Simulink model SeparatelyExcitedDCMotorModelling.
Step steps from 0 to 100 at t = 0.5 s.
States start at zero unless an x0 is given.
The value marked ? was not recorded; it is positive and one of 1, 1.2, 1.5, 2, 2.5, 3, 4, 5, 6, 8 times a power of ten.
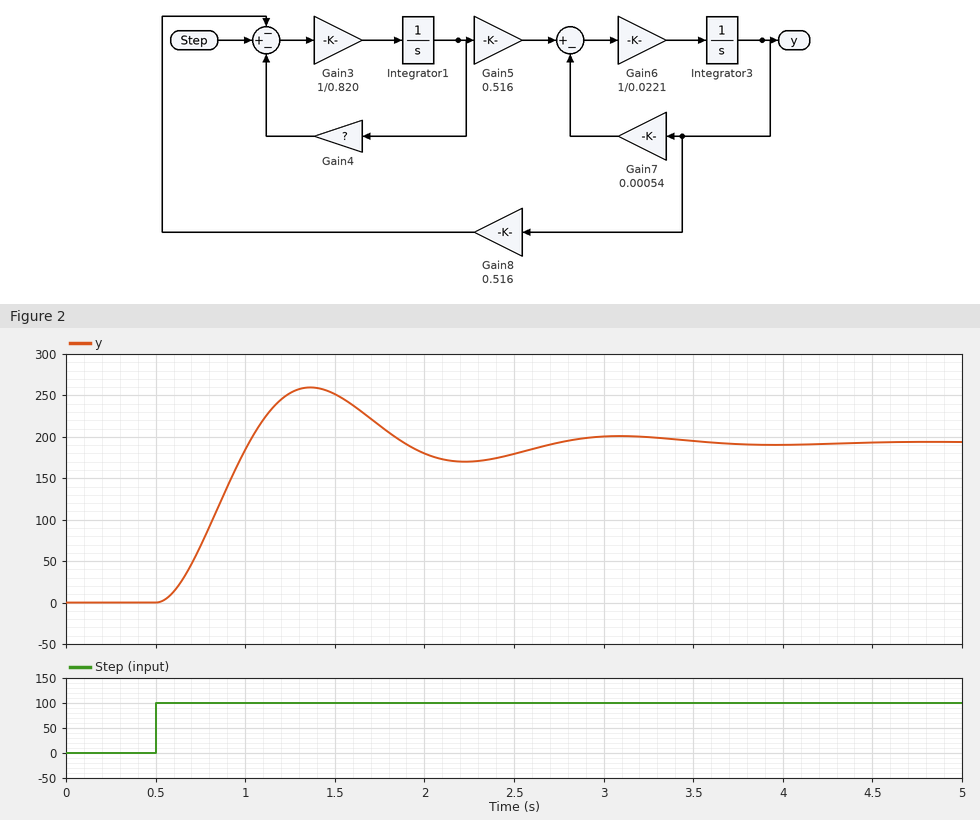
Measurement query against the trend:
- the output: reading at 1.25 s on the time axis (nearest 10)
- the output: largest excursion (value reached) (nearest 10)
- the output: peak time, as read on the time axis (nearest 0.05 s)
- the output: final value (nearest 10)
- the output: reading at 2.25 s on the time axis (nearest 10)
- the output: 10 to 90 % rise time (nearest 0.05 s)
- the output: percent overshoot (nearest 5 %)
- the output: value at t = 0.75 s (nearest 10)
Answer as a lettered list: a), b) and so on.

a) 250
b) 260
c) 1.35 s
d) 190
e) 170
f) 0.35 s
g) 35 %
h) 70
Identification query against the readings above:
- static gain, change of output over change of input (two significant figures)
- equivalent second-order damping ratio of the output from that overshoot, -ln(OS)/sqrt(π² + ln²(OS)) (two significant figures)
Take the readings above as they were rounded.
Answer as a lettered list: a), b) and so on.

a) 1.9
b) 0.32
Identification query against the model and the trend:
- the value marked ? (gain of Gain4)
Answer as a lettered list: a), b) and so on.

a) 2
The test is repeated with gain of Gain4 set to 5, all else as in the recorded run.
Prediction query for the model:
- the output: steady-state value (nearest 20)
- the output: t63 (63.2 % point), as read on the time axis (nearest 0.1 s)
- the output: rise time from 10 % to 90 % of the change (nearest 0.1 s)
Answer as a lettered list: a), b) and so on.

a) 200
b) 1.0 s
c) 0.6 s
